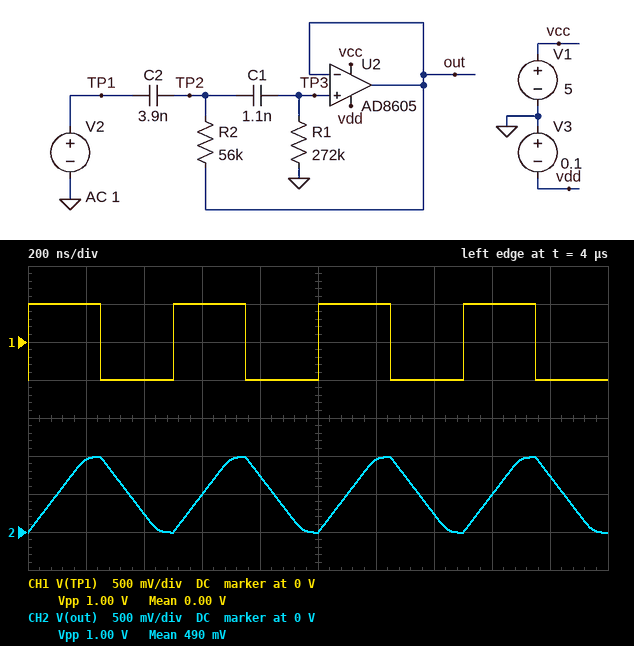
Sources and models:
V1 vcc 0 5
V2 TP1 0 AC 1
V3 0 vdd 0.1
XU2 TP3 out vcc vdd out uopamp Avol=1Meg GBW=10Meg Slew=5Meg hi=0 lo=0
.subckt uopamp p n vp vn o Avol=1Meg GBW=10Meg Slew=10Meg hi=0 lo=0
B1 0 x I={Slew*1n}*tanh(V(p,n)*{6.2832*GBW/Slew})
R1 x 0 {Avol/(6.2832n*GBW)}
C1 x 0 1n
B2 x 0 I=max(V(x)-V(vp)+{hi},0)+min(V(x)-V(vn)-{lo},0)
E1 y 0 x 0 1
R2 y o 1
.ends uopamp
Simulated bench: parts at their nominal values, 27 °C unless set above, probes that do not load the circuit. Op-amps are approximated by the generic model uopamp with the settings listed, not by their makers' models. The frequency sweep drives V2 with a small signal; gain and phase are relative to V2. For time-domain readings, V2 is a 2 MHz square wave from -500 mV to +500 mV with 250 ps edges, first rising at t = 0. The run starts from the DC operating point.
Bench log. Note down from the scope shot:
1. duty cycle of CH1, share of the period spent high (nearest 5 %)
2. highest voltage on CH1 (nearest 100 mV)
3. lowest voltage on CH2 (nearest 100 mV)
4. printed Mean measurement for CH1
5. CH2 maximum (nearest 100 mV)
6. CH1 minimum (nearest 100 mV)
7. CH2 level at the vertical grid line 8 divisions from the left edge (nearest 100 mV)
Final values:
50 %
500 mV
0 V
0.00 V
1.0 V
-500 mV
500 mV
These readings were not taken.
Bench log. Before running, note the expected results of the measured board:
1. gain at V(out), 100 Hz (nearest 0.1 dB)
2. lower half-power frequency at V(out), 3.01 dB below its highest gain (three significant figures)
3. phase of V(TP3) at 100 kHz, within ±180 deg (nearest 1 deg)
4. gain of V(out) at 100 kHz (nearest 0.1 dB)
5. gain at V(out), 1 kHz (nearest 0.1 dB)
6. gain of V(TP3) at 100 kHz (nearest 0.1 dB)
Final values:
-31.7 dB
543 Hz
0 deg
0 dB
0.8 dB
0 dB
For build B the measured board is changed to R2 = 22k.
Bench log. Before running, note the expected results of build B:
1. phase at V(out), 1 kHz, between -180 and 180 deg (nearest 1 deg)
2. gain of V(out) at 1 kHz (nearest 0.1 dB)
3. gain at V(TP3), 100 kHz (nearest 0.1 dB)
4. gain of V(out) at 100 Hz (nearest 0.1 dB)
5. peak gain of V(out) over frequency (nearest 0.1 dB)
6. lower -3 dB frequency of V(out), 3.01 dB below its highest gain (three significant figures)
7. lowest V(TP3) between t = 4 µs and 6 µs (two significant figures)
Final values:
89 deg
3.3 dB
0 dB
-39.8 dB
3.8 dB
837 Hz
-14 mV
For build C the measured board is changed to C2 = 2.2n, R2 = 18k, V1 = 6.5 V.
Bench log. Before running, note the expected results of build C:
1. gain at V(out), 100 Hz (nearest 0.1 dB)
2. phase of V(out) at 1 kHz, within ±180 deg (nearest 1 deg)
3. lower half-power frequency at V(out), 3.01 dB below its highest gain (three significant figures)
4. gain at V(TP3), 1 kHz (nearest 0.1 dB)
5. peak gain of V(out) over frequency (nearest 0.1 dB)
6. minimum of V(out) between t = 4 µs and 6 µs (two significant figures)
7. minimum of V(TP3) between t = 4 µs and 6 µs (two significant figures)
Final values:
-46.6 dB
145 deg
1.25 kHz
-2.9 dB
5.6 dB
-14 mV
-18 mV
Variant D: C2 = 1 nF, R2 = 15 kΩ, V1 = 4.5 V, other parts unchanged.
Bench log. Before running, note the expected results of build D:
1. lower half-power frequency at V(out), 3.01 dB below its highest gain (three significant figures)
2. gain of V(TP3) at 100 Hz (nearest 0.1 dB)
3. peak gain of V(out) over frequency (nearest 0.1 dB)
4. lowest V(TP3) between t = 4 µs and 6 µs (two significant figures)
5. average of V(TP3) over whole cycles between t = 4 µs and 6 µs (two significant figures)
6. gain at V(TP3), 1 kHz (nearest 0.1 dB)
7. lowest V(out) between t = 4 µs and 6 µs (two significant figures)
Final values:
2.05 kHz
-55.0 dB
6.8 dB
-29 mV
480 mV
-13.6 dB
-21 mV
